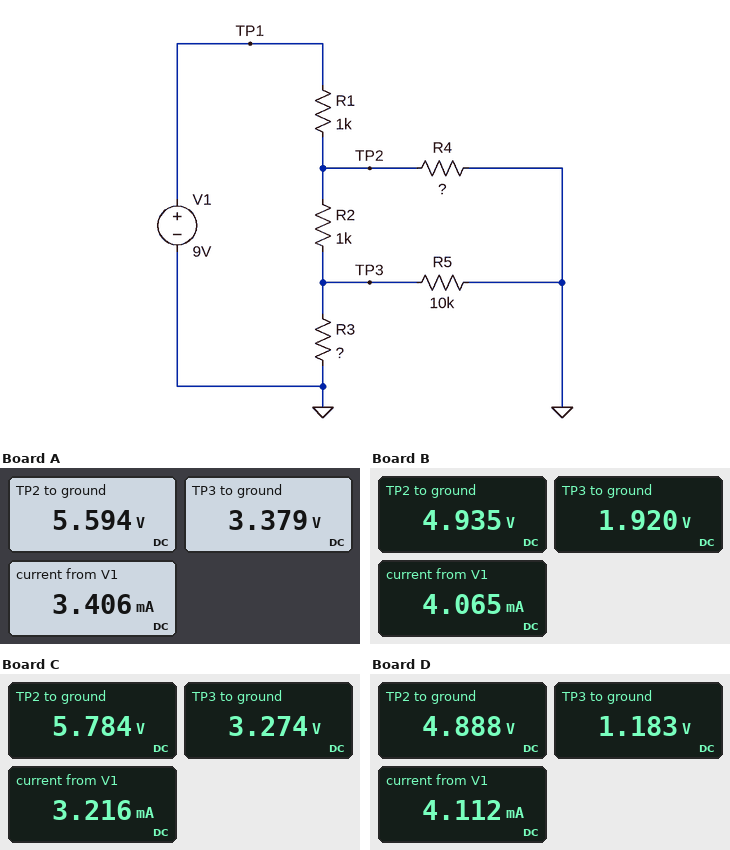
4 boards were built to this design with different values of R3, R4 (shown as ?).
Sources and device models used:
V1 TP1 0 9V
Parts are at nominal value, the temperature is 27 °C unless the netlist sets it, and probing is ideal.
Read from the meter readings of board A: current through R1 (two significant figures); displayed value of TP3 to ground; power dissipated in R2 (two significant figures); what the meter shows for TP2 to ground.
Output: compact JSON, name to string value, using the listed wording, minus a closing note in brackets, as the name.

{"current through R1": "3.4 mA", "displayed value of TP3 to ground": "3.379 V", "power dissipated in R2": "4.9 mW", "what the meter shows for TP2 to ground": "5.594 V"}
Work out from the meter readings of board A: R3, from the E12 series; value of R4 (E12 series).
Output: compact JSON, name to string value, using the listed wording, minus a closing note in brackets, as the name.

{"R3, from the E12 series": "1.8 kΩ", "value of R4": "4.7 kΩ"}
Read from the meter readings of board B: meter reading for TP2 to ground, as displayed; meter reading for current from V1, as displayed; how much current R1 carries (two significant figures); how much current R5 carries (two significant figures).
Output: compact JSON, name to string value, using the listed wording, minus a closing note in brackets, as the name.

{"meter reading for TP2 to ground, as displayed": "4.935 V", "meter reading for current from V1, as displayed": "4.065 mA", "how much current R1 carries": "4.1 mA", "how much current R5 carries": "190 µA"}
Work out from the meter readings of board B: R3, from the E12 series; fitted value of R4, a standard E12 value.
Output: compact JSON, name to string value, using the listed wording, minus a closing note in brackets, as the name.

{"R3, from the E12 series": "680 Ω", "fitted value of R4, a standard E12 value": "4.7 kΩ"}
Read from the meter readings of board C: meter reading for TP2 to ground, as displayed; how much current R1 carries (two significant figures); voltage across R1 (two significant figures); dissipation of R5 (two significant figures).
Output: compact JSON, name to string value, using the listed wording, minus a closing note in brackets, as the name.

{"meter reading for TP2 to ground, as displayed": "5.784 V", "how much current R1 carries": "3.2 mA", "voltage across R1": "3.2 V", "dissipation of R5": "1.1 mW"}
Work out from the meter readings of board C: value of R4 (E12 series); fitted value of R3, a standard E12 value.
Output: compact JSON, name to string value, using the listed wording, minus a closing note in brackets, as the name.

{"value of R4": "8.2 kΩ", "fitted value of R3, a standard E12 value": "1.5 kΩ"}
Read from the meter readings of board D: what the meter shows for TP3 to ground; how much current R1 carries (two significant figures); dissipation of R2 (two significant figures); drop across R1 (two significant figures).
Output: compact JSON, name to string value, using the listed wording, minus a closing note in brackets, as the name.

{"what the meter shows for TP3 to ground": "1.183 V", "how much current R1 carries": "4.1 mA", "dissipation of R2": "14 mW", "drop across R1": "4.1 V"}
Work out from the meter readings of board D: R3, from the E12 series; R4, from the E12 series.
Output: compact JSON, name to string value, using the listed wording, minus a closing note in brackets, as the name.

{"R3, from the E12 series": "330 Ω", "R4, from the E12 series": "12 kΩ"}
